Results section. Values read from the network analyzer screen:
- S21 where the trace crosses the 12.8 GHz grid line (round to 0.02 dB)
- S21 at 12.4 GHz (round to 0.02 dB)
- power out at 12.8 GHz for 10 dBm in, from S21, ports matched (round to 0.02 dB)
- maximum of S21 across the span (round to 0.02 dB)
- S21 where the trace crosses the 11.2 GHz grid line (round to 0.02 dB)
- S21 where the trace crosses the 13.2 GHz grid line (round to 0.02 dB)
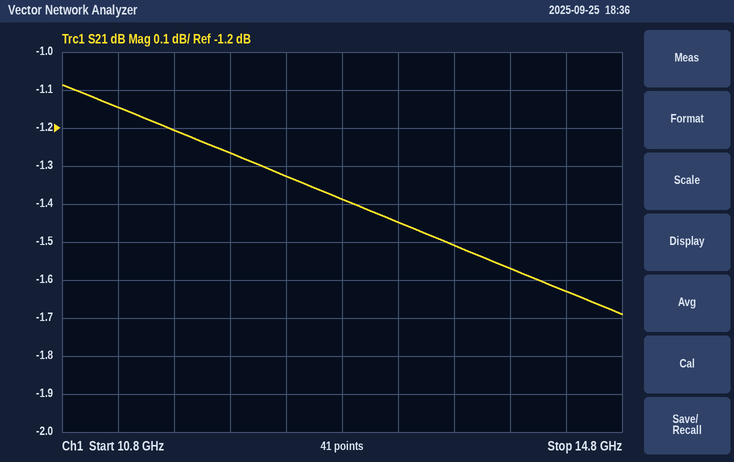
-1.38 dB
-1.32 dB
8.62 dBm
-1.08 dB
-1.14 dB
-1.44 dB
